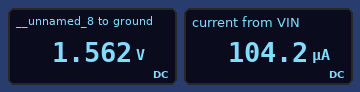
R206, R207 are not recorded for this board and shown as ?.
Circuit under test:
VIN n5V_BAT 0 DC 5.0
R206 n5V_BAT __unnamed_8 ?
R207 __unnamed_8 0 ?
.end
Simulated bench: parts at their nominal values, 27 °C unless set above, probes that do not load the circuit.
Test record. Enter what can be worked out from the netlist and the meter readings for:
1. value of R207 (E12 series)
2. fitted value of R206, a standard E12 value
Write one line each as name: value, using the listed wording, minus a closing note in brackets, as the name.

value of R207: 15 kΩ
fitted value of R206, a standard E12 value: 33 kΩ
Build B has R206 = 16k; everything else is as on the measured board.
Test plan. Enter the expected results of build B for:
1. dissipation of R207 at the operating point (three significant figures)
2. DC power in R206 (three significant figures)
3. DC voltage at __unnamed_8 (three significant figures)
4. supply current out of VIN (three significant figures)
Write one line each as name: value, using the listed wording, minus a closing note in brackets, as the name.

dissipation of R207 at the operating point: 390 µW
DC power in R206: 416 µW
DC voltage at __unnamed_8: 2.42 V
supply current out of VIN: 161 µA
